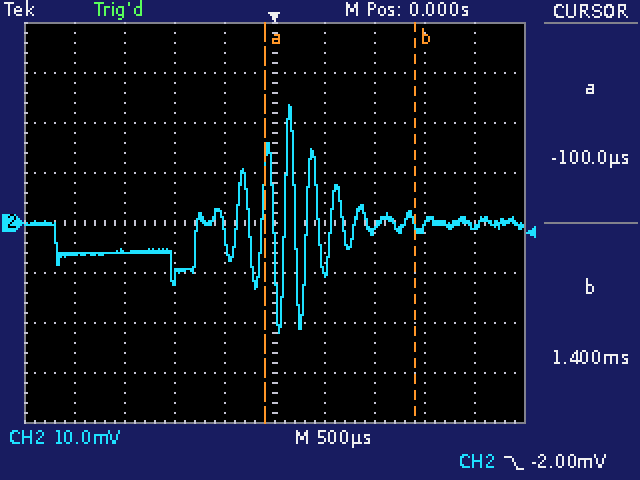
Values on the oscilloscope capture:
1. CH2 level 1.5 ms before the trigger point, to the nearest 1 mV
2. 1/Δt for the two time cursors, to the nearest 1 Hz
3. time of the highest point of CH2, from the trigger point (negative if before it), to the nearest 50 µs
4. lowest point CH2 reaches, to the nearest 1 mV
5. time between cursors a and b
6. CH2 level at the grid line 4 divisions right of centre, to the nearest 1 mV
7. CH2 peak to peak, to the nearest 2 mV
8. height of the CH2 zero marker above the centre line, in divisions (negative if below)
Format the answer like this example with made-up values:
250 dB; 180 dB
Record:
-6 mV; 667 Hz; +150 µs; -22 mV; 1.50 ms; -1 mV; 46 mV; 0.0 div
